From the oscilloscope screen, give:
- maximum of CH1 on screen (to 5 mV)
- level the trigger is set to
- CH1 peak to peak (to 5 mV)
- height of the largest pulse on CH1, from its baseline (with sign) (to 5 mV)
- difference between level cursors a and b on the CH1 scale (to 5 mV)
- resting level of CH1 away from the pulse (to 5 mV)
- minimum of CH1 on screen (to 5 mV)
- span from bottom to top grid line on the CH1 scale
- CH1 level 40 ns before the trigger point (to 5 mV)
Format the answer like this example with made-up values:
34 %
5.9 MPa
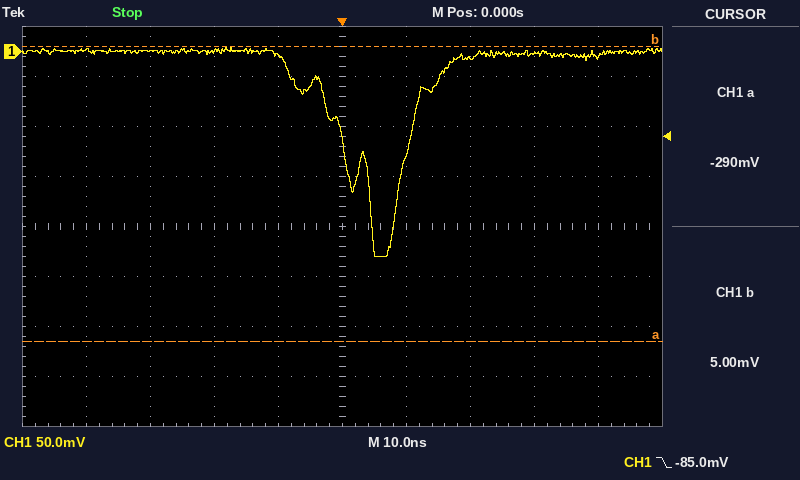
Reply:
5 mV
-85.0 mV
210 mV
-205 mV
295 mV
0 mV
-205 mV
400 mV
0 mV
